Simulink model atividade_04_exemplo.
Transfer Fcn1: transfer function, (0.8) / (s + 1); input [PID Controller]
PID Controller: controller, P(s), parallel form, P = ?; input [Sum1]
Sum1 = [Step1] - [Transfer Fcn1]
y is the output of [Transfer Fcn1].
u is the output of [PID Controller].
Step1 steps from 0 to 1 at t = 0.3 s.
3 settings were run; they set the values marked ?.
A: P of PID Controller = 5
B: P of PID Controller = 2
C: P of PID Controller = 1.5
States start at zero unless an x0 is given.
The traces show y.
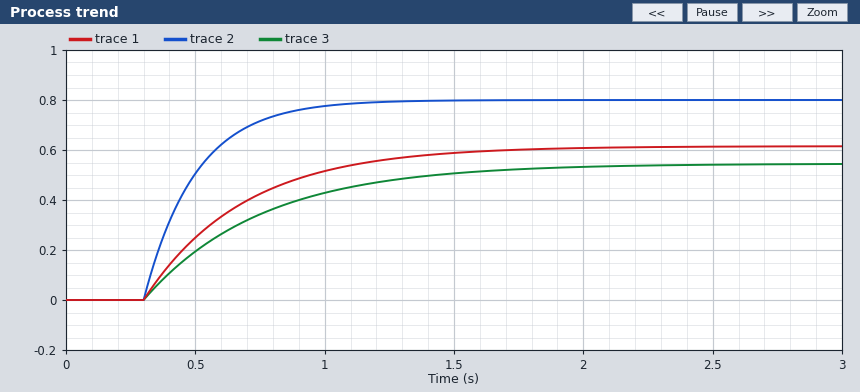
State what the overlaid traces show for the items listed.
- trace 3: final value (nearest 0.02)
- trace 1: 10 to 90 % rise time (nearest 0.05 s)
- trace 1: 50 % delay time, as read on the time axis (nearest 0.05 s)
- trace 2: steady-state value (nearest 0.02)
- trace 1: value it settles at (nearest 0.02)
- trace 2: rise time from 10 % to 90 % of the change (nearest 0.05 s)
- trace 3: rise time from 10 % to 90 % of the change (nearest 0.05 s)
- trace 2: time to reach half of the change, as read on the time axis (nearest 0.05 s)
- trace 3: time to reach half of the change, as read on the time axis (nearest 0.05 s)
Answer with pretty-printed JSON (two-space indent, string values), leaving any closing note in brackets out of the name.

{
  "trace 3: final value": "0.54",
  "trace 1: 10 to 90 % rise time": "0.85 s",
  "trace 1: 50 % delay time, as read on the time axis": "0.55 s",
  "trace 2: steady-state value": "0.80",
  "trace 1: value it settles at": "0.62",
  "trace 2: rise time from 10 % to 90 % of the change": "0.45 s",
  "trace 3: rise time from 10 % to 90 % of the change": "1.00 s",
  "trace 2: time to reach half of the change, as read on the time axis": "0.45 s",
  "trace 3: time to reach half of the change, as read on the time axis": "0.60 s"
}
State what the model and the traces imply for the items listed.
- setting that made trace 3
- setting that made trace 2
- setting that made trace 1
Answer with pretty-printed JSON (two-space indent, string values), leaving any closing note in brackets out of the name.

{
  "setting that made trace 3": "C",
  "setting that made trace 2": "A",
  "setting that made trace 1": "B"
}
